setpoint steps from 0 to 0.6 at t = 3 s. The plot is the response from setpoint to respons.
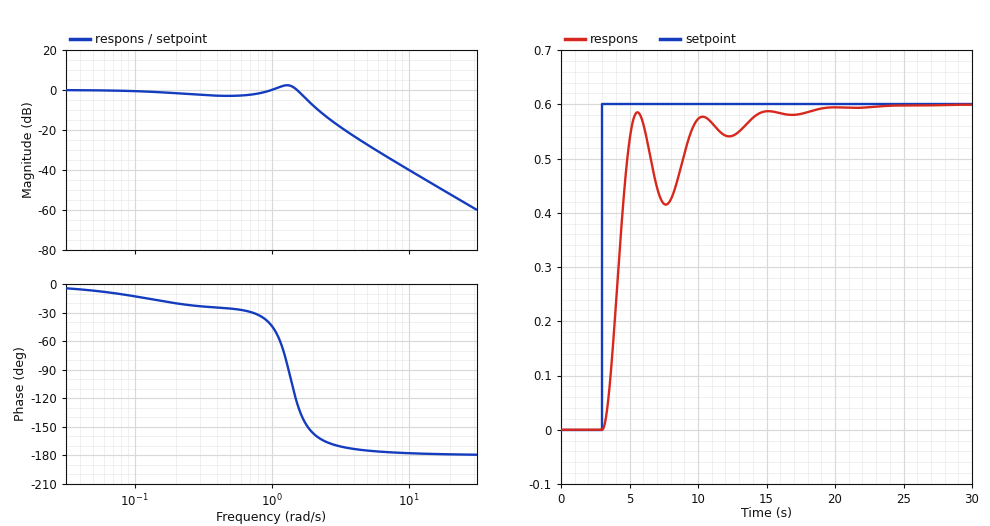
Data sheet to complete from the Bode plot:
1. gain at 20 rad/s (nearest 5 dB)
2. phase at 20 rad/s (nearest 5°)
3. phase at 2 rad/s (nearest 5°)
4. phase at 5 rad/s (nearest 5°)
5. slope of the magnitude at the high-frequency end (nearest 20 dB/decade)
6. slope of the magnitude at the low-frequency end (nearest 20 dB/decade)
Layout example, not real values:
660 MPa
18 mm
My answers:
-50 dB
-180°
-155°
-175°
-40 dB/decade
0 dB/decade
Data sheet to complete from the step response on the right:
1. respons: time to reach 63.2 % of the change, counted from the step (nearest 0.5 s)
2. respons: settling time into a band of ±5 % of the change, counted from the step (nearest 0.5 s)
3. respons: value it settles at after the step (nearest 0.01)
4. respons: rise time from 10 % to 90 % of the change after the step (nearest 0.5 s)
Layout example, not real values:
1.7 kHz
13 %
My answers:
1.5 s
11.0 s
0.60
1.5 s
